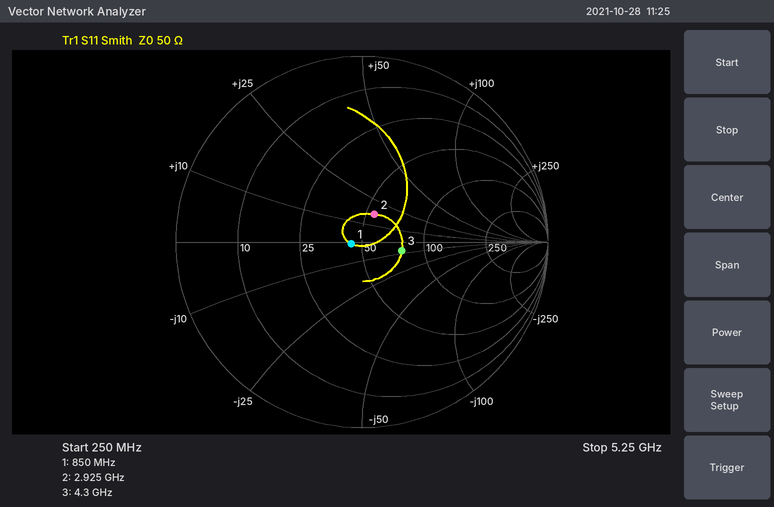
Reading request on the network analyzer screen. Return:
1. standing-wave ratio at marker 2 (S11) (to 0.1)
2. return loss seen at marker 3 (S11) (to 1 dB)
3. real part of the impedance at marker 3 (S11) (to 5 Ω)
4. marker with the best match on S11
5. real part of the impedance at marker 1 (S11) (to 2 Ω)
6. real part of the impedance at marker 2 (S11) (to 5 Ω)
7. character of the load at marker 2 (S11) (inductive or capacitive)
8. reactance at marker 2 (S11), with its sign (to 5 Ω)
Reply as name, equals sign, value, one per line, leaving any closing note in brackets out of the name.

standing-wave ratio at marker 2 (S11) = 1.4
return loss seen at marker 3 (S11) = 13 dB
real part of the impedance at marker 3 (S11) = 75 Ω
marker with the best match on S11 = marker 1
real part of the impedance at marker 1 (S11) = 44 Ω
real part of the impedance at marker 2 (S11) = 55 Ω
character of the load at marker 2 (S11) = inductive
reactance at marker 2 (S11), with its sign = +15 Ω
